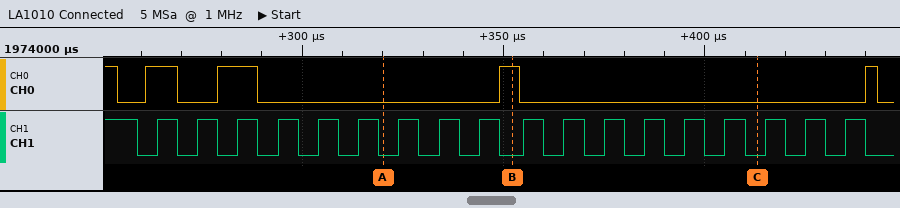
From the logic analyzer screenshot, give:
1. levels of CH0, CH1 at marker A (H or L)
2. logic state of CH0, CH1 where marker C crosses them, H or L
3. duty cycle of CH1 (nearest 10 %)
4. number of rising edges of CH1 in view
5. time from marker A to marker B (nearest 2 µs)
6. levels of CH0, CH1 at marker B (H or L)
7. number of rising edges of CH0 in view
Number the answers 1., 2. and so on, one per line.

1. CH0=L, CH1=L
2. CH0=L, CH1=L
3. 50 %
4. 18
5. 32 µs
6. CH0=H, CH1=L
7. 4
